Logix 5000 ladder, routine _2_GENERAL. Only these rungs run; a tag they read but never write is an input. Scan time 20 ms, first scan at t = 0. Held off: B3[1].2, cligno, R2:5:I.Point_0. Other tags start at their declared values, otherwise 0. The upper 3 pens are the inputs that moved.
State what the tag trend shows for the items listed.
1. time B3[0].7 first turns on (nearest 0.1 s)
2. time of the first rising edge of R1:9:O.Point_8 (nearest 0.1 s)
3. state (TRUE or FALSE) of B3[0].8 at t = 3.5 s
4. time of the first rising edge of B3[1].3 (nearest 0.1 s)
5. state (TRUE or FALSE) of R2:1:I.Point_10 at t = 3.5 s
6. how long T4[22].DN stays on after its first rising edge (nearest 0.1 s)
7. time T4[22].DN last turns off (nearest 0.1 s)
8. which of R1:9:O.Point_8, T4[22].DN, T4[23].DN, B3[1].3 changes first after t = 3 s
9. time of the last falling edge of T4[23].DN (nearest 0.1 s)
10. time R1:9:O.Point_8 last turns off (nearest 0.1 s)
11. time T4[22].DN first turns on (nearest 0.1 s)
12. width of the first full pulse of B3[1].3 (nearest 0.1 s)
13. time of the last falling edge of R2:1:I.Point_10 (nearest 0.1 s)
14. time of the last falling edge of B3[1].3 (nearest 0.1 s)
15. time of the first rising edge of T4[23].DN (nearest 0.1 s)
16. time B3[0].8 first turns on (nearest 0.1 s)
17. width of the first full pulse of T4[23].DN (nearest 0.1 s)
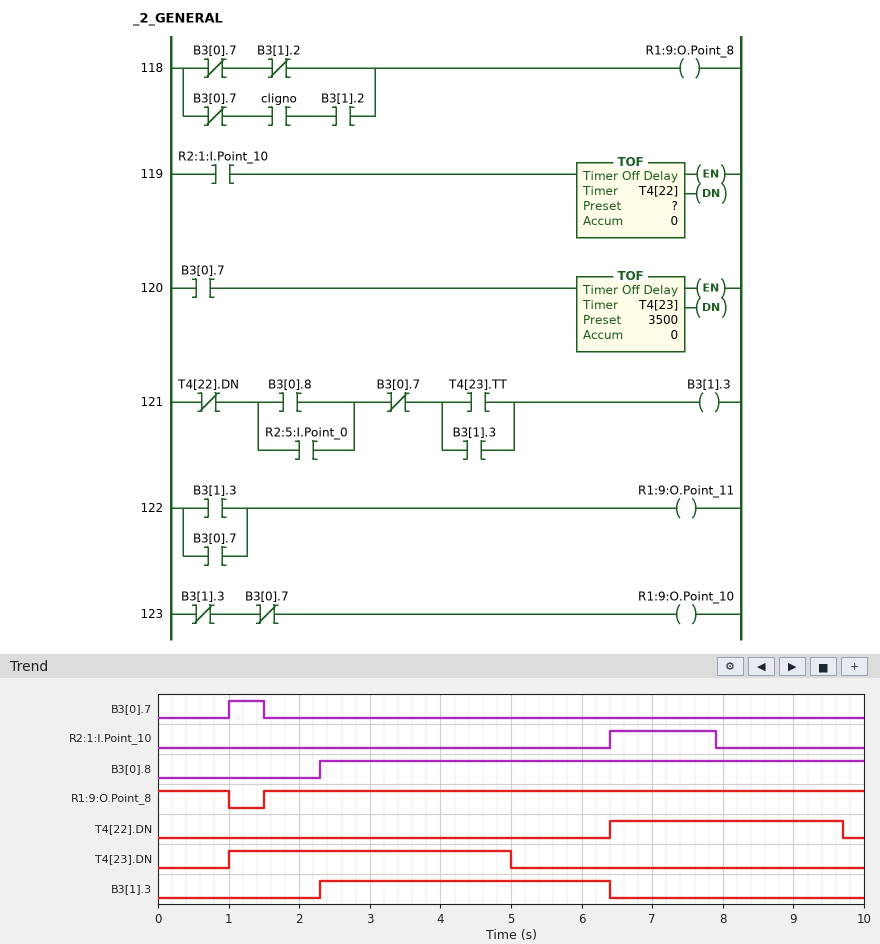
1.0 s
1.5 s
TRUE
2.3 s
FALSE
3.3 s
9.7 s
T4[23].DN
5.0 s
1.0 s
6.4 s
4.1 s
7.9 s
6.4 s
1.0 s
2.3 s
4.0 s
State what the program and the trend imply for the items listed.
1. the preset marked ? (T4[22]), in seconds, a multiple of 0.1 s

1.8 s
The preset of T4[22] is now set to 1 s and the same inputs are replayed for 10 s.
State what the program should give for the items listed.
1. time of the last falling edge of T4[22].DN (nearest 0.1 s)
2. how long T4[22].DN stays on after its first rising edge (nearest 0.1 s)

8.9 s
2.5 s
